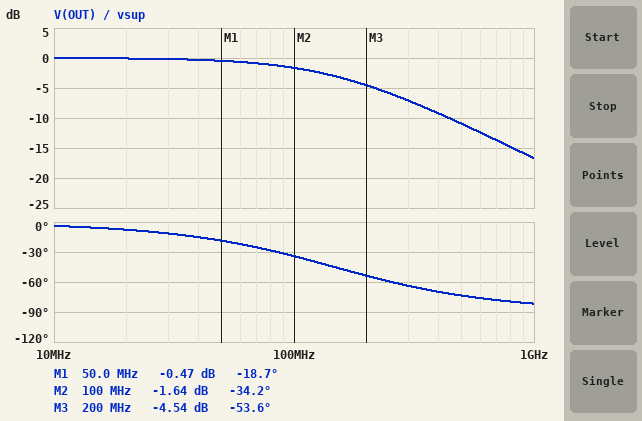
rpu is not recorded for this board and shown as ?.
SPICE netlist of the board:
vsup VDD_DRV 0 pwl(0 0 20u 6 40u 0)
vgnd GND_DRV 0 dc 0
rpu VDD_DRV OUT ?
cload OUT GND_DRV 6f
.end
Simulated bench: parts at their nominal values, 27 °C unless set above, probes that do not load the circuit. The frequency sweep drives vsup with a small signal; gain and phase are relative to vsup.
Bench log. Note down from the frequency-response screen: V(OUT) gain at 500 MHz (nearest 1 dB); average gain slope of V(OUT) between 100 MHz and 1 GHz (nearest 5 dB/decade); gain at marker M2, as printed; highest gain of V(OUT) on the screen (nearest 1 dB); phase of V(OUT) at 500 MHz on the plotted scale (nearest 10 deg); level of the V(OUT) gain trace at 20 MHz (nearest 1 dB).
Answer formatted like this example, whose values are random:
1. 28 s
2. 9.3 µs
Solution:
1. -11 dB
2. -15 dB/decade
3. -1.64 dB
4. 0 dB
5. -70 deg
6. 0 dB
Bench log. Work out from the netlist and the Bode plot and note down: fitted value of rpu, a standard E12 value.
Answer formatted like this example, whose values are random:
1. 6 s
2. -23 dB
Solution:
1. 180 kΩ
